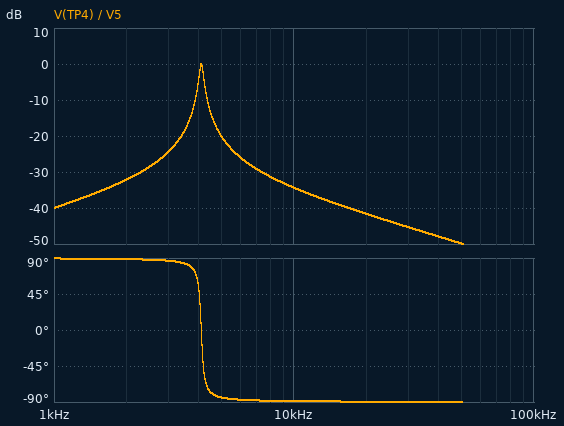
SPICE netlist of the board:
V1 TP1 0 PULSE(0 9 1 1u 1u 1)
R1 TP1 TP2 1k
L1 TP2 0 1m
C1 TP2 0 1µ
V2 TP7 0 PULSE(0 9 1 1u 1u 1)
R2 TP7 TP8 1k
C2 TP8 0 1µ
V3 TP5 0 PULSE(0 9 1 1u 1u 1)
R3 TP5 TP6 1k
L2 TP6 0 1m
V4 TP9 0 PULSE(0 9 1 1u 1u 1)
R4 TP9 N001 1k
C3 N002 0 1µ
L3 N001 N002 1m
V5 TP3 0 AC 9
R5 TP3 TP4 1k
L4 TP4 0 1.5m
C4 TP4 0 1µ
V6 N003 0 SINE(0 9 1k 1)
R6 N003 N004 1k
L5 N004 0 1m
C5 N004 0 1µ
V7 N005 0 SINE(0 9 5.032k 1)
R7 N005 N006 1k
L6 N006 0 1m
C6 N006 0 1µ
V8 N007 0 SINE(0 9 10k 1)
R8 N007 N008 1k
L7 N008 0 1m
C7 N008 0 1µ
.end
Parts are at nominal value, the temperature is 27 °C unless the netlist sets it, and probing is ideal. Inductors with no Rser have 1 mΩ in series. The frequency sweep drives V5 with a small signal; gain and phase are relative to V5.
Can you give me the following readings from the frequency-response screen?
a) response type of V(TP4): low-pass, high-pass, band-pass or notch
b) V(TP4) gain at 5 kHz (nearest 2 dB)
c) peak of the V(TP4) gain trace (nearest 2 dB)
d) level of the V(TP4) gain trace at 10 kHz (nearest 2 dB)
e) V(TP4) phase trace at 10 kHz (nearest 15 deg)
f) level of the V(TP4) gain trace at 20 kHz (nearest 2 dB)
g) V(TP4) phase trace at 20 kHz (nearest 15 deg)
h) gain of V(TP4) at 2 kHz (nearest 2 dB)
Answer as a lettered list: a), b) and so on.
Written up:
a) band-pass
b) -20 dB
c) 0 dB
d) -34 dB
e) -90 deg
f) -42 dB
g) -90 deg
h) -32 dB
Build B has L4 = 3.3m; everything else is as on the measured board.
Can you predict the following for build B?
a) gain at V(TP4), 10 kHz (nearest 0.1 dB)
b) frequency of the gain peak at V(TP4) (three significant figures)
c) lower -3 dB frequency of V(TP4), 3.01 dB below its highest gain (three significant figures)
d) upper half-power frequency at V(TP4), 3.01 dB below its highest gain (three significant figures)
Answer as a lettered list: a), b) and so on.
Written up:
a) -35.3 dB
b) 2.77 kHz
c) 2.69 kHz
d) 2.85 kHz
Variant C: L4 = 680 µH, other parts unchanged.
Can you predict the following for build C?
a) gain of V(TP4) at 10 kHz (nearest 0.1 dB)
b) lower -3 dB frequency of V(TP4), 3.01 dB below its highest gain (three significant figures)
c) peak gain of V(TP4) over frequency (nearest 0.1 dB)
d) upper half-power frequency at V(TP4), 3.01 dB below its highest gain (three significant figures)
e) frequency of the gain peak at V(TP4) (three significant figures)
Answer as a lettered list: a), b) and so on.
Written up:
a) -31.9 dB
b) 6.02 kHz
c) 0 dB
d) 6.18 kHz
e) 6.10 kHz
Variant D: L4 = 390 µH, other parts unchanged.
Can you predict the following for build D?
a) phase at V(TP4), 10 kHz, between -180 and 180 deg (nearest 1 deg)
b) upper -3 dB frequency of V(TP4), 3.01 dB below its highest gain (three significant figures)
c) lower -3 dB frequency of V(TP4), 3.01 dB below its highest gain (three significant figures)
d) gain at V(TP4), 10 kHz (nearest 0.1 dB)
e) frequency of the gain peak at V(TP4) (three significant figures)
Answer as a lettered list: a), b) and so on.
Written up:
a) -87 deg
b) 8.14 kHz
c) 7.98 kHz
d) -26.9 dB
e) 8.06 kHz
